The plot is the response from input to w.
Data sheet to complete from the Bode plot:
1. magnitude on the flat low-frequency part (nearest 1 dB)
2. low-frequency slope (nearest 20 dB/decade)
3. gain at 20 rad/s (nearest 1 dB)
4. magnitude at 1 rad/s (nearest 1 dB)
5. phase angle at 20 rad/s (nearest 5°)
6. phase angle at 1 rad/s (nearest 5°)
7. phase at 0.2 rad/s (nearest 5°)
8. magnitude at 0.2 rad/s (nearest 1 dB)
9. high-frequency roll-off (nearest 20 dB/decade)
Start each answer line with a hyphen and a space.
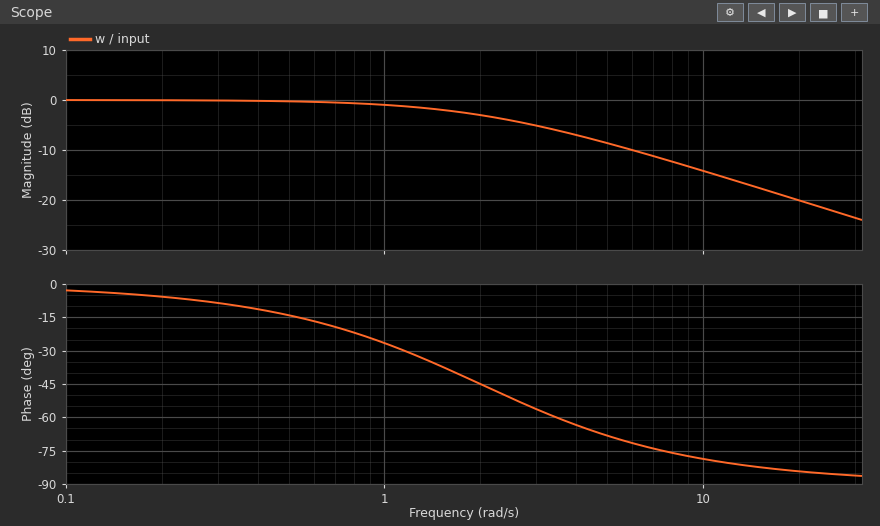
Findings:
- 0 dB
- 0 dB/decade
- -20 dB
- -1 dB
- -85°
- -25°
- -5°
- 0 dB
- -20 dB/decade
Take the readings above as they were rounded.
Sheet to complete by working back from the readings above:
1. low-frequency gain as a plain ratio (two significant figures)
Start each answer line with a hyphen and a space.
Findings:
- 1.0
